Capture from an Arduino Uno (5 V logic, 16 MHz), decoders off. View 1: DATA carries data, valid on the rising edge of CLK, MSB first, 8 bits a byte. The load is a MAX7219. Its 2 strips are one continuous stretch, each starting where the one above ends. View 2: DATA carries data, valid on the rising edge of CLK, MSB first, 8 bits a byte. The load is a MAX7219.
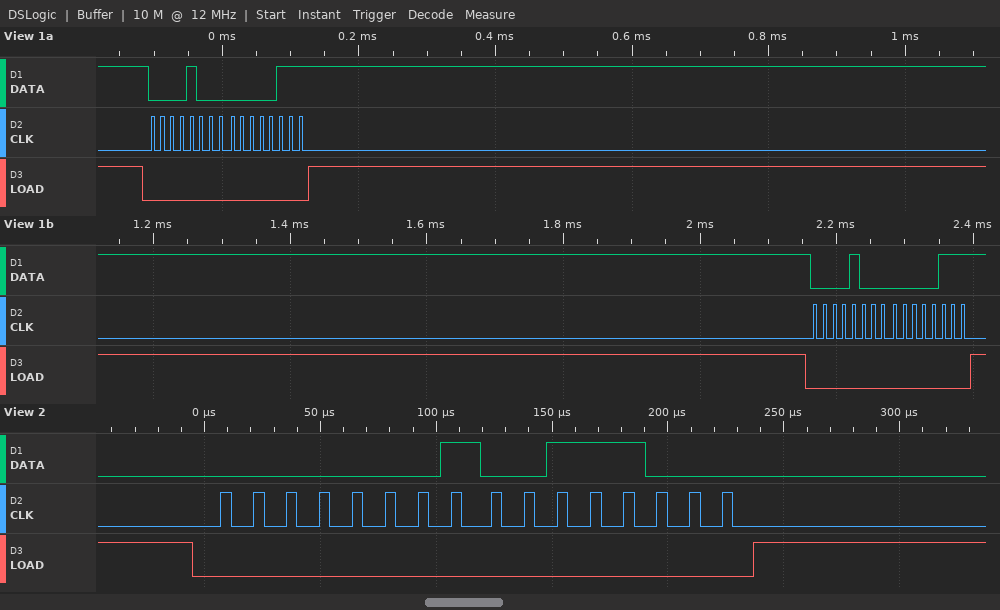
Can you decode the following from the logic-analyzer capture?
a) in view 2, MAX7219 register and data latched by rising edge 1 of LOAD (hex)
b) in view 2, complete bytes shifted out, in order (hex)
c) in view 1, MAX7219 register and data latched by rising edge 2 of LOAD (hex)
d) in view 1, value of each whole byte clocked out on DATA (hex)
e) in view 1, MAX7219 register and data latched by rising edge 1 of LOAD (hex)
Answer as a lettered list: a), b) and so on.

a) register 0x1, data 0x38
b) 01 38
c) register 0x8, data 0x07
d) 08 07 08 07
e) register 0x8, data 0x07
